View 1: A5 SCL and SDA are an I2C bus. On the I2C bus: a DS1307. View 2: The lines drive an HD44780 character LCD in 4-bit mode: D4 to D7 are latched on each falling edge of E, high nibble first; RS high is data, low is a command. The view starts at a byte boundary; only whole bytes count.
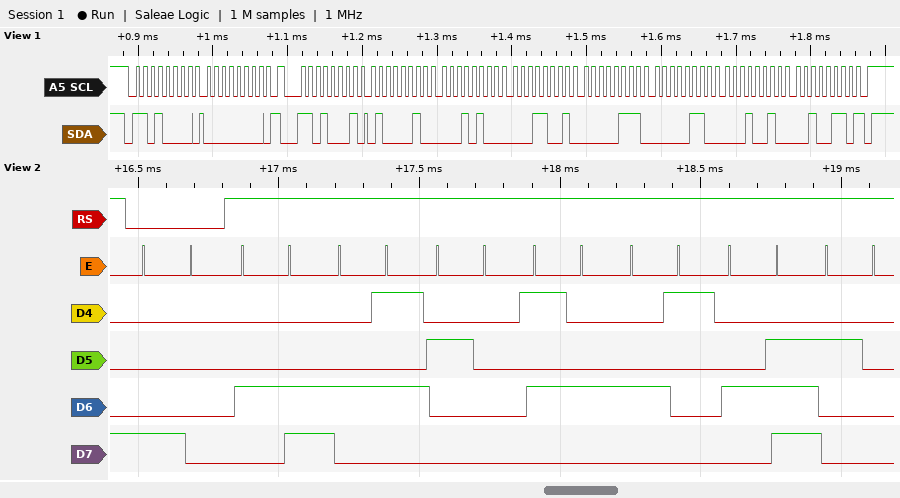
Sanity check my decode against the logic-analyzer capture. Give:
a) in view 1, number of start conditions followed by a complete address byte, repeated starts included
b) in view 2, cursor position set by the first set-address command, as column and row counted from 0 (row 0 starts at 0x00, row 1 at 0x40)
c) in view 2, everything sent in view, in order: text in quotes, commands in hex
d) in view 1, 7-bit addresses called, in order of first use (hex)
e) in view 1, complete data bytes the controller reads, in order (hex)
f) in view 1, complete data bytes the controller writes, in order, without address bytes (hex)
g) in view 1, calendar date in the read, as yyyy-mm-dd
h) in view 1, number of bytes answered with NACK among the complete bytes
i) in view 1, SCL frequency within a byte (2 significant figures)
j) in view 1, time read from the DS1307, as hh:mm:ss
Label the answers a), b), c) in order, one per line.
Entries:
a) 2
b) column 0, row 0
c) 0x80 "LE TAN "
d) 0x68
e) 42 14 19 07 06 12 26
f) 00
g) 2026-12-06
h) 1
i) 100 kHz
j) 19:14:42
